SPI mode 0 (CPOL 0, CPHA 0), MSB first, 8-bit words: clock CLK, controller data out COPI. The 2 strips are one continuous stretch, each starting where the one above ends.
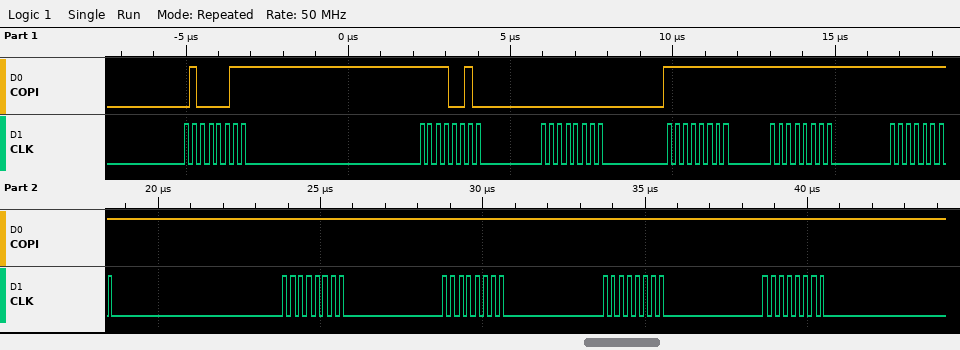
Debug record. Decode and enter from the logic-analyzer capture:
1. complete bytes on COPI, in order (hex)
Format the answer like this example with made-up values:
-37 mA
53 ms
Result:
43 F2 00 FF FF FF FF FF FF FF
